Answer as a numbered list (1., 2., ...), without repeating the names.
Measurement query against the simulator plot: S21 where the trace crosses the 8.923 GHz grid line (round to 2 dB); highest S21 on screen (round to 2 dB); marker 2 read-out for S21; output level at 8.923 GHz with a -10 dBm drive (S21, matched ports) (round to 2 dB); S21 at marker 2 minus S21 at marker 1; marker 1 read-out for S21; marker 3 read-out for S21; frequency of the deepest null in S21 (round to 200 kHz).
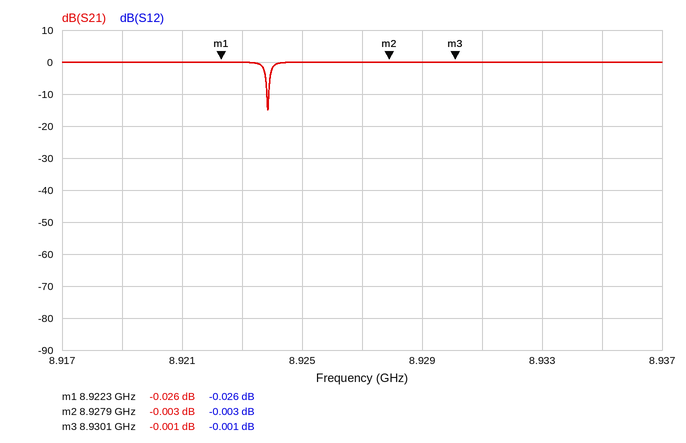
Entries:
1. 0 dB
2. 0 dB
3. -0.003 dB
4. -10 dBm
5. 0.023 dB
6. -0.026 dB
7. -0.001 dB
8. 8.9238 GHz
